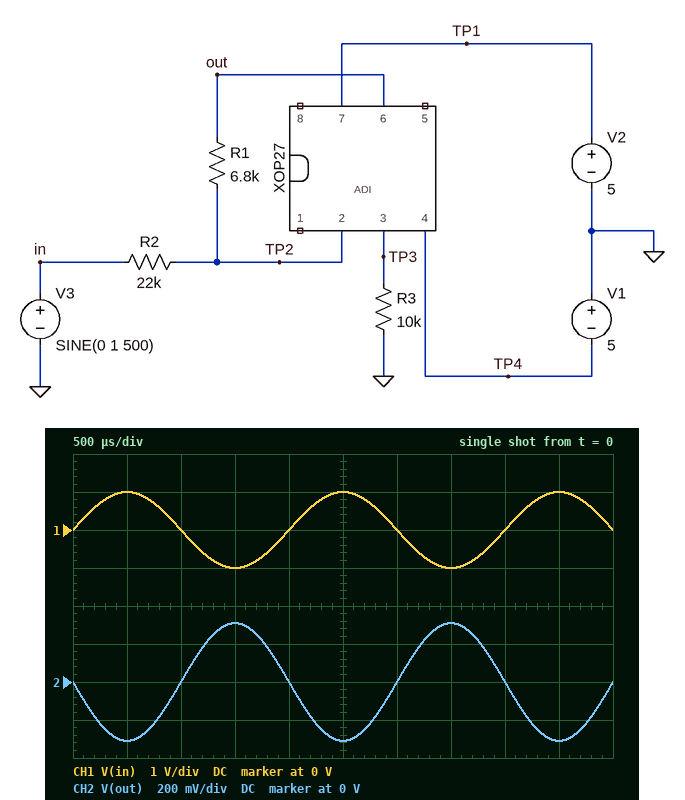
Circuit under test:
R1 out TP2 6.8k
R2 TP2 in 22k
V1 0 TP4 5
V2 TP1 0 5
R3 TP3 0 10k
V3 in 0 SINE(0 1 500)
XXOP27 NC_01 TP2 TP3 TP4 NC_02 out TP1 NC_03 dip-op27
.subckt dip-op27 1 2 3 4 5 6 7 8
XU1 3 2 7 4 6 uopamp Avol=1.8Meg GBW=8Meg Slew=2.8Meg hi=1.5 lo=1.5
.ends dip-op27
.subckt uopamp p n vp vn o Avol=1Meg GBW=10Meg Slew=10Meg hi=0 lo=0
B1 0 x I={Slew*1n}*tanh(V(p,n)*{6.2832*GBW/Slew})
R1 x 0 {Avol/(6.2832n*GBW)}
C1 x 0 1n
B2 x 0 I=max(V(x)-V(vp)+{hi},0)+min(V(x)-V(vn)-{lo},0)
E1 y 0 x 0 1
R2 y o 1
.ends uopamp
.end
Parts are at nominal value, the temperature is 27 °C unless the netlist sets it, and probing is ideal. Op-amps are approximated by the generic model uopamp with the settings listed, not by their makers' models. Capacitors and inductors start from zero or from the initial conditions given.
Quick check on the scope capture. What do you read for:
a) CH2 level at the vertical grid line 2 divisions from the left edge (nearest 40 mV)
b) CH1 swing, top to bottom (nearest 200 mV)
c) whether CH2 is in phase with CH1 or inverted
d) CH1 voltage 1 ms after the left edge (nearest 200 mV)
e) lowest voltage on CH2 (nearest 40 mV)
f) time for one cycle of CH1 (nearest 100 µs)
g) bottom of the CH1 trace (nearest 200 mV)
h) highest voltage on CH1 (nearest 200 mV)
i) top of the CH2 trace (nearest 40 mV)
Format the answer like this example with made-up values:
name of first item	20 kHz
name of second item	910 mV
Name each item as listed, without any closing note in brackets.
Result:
CH2 level at the vertical grid line 2 divisions from the left edge	0 V
CH1 swing, top to bottom	2.0 V
whether CH2 is in phase with CH1 or inverted	inverted
CH1 voltage 1 ms after the left edge	0 V
lowest voltage on CH2	-320 mV
time for one cycle of CH1	2.0 ms
bottom of the CH1 trace	-1.0 V
highest voltage on CH1	1.0 V
top of the CH2 trace	320 mV
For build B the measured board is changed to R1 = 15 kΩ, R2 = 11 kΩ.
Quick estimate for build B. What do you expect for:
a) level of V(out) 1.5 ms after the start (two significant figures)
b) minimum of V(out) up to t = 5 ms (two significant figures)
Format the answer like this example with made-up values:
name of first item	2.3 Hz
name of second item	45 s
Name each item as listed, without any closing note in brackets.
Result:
level of V(out) 1.5 ms after the start	1.4 V
minimum of V(out) up to t = 5 ms	-1.4 V
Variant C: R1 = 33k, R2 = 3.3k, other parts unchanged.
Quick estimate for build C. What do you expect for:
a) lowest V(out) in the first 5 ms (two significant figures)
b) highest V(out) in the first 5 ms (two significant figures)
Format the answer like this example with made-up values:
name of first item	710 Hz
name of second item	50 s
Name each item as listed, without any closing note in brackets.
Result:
lowest V(out) in the first 5 ms	-3.5 V
highest V(out) in the first 5 ms	3.5 V
